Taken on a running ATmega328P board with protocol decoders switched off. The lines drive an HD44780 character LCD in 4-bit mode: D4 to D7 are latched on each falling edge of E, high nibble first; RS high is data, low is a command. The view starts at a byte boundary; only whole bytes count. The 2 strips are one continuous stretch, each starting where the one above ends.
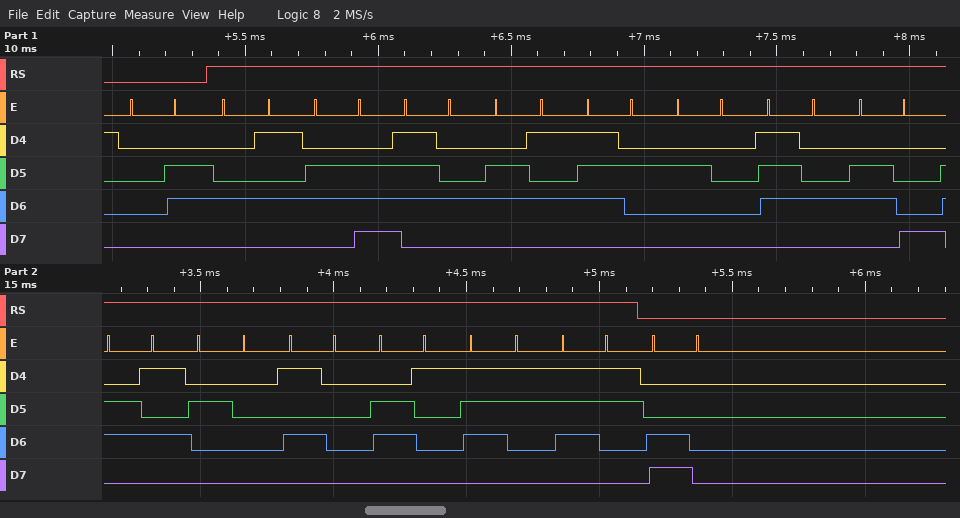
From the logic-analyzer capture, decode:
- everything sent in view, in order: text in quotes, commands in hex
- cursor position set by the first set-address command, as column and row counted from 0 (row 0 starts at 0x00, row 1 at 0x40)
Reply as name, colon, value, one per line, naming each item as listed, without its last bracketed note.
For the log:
everything sent in view, in order: text in quotes, commands in hex: 0x06 "Enter the Pass" 0xC0
cursor position set by the first set-address command, as column and row counted from 0: column 0, row 1
